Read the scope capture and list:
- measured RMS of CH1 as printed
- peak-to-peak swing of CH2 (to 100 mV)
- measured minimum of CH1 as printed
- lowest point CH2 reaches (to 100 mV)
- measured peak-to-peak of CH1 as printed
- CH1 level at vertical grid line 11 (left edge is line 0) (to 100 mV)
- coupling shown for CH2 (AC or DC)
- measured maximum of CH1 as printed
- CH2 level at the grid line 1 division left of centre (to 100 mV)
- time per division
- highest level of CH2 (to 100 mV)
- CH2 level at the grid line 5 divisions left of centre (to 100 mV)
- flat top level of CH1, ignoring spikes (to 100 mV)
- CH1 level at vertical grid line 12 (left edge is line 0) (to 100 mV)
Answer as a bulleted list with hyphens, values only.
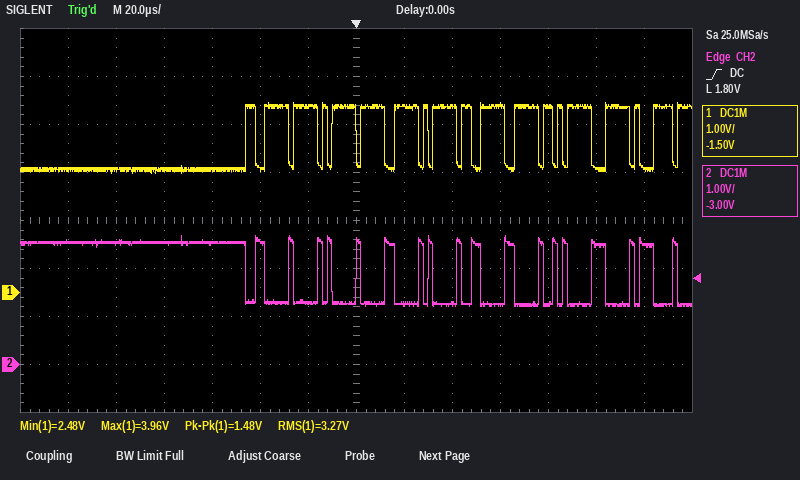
- 3.27 V
- 1.5 V
- 2.48 V
- 1.2 V
- 1.48 V
- 3.9 V
- DC
- 3.96 V
- 1.3 V
- 20 µs
- 2.7 V
- 2.5 V
- 3.9 V
- 2.6 V
